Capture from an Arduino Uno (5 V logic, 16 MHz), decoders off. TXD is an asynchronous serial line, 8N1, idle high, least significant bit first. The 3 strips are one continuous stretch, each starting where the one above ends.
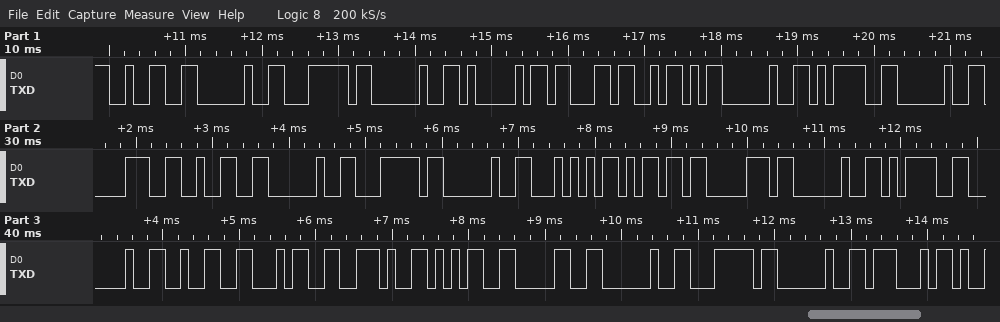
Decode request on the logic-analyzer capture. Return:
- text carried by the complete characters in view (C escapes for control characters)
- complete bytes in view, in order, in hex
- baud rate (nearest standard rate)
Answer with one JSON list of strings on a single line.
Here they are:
["\"2 | AcZ = 82 | Tmp = 24.50 | G\"", "0x32 0x20 0x7C 0x20 0x41 0x63 0x5A 0x20 0x3D 0x20 0x38 0x32 0x20 0x7C 0x20 0x54 0x6D 0x70 0x20 0x3D 0x20 0x32 0x34 0x2E 0x35 0x30 0x20 0x7C 0x20 0x47", "9600 baud"]
